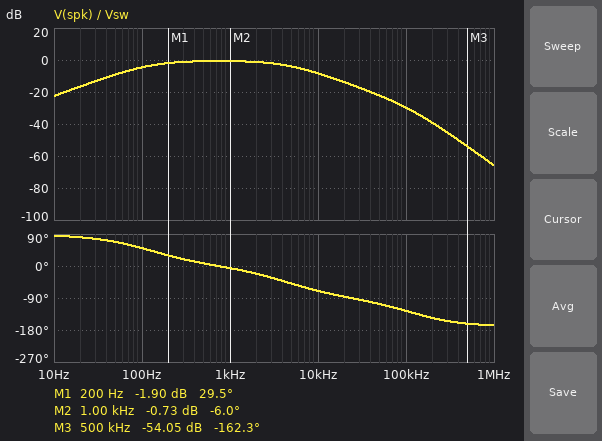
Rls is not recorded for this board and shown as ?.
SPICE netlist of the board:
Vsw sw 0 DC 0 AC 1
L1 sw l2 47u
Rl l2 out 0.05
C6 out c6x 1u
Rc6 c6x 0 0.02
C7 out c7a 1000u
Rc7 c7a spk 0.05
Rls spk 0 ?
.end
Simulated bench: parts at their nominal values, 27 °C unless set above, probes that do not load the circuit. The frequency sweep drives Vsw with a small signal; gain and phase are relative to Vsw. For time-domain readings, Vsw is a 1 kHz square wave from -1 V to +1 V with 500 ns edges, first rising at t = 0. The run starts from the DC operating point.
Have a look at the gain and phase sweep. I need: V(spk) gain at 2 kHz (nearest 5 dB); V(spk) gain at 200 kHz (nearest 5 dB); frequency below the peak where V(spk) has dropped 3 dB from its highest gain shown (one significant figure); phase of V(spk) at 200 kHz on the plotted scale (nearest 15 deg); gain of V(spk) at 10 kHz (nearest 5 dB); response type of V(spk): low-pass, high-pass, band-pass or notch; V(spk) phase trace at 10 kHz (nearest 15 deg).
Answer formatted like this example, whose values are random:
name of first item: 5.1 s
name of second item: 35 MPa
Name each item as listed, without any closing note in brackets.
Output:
V(spk) gain at 2 kHz: 0 dB
V(spk) gain at 200 kHz: -40 dB
frequency below the peak where V(spk) has dropped 3 dB from its highest gain shown: 100 Hz
phase of V(spk) at 200 kHz on the plotted scale: -150 deg
gain of V(spk) at 10 kHz: -10 dB
response type of V(spk): low-pass, high-pass, band-pass or notch: band-pass
V(spk) phase trace at 10 kHz: -75 deg
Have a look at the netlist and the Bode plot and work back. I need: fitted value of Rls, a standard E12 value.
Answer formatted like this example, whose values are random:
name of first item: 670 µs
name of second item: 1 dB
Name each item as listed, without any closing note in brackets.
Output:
fitted value of Rls, a standard E12 value: 1.2 Ω
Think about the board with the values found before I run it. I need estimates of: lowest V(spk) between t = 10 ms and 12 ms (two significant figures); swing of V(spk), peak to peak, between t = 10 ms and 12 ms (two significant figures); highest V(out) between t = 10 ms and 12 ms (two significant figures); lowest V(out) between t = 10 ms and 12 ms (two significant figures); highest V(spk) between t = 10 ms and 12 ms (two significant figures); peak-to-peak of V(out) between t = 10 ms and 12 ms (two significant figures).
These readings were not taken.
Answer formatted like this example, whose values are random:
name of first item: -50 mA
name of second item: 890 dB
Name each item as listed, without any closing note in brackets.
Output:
lowest V(spk) between t = 10 ms and 12 ms: -1.0 V
swing of V(spk), peak to peak, between t = 10 ms and 12 ms: 2.0 V
highest V(out) between t = 10 ms and 12 ms: 990 mV
lowest V(out) between t = 10 ms and 12 ms: -990 mV
highest V(spk) between t = 10 ms and 12 ms: 1.0 V
peak-to-peak of V(out) between t = 10 ms and 12 ms: 2.0 V
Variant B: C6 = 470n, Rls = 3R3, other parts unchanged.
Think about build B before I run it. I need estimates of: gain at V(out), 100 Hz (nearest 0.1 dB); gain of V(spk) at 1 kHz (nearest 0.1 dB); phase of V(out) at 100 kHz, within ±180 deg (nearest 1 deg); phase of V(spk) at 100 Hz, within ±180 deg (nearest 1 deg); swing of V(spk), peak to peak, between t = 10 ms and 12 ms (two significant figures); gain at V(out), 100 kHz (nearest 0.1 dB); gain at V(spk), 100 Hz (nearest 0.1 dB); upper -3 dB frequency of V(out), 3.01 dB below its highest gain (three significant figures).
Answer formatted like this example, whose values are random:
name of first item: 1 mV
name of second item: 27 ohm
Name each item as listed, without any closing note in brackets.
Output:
gain at V(out), 100 Hz: -0.1 dB
gain of V(spk) at 1 kHz: -0.3 dB
phase of V(out) at 100 kHz, within ±180 deg: -131 deg
phase of V(spk) at 100 Hz, within ±180 deg: 25 deg
swing of V(spk), peak to peak, between t = 10 ms and 12 ms: 2.1 V
gain at V(out), 100 kHz: -21.4 dB
gain at V(spk), 100 Hz: -1.1 dB
upper -3 dB frequency of V(out), 3.01 dB below its highest gain: 12.6 kHz
